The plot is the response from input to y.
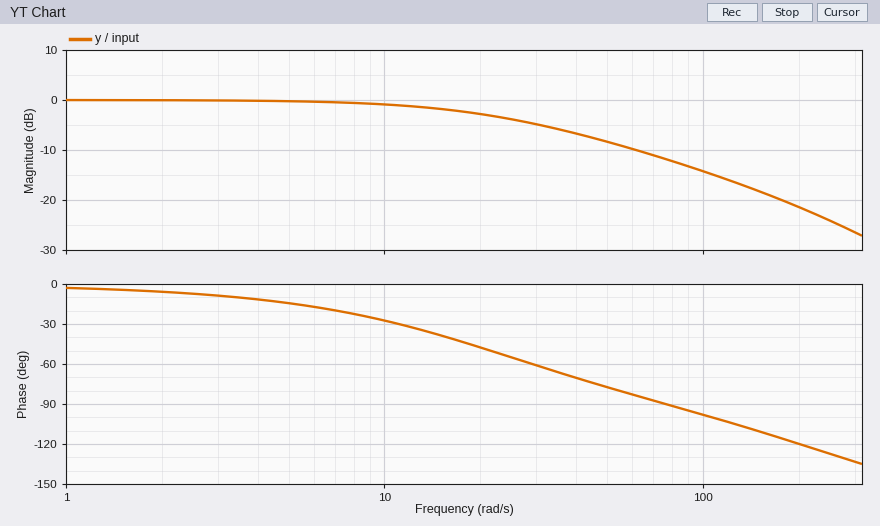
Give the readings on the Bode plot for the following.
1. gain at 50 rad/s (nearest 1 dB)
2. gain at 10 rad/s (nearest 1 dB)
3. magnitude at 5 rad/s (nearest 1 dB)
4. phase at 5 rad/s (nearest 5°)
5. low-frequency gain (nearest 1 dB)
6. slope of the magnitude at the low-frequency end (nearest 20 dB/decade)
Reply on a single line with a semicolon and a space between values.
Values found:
-8 dB; -1 dB; 0 dB; -15°; 0 dB; 0 dB/decade
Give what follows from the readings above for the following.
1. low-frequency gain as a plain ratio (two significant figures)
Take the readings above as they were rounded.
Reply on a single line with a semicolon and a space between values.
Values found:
1.0
